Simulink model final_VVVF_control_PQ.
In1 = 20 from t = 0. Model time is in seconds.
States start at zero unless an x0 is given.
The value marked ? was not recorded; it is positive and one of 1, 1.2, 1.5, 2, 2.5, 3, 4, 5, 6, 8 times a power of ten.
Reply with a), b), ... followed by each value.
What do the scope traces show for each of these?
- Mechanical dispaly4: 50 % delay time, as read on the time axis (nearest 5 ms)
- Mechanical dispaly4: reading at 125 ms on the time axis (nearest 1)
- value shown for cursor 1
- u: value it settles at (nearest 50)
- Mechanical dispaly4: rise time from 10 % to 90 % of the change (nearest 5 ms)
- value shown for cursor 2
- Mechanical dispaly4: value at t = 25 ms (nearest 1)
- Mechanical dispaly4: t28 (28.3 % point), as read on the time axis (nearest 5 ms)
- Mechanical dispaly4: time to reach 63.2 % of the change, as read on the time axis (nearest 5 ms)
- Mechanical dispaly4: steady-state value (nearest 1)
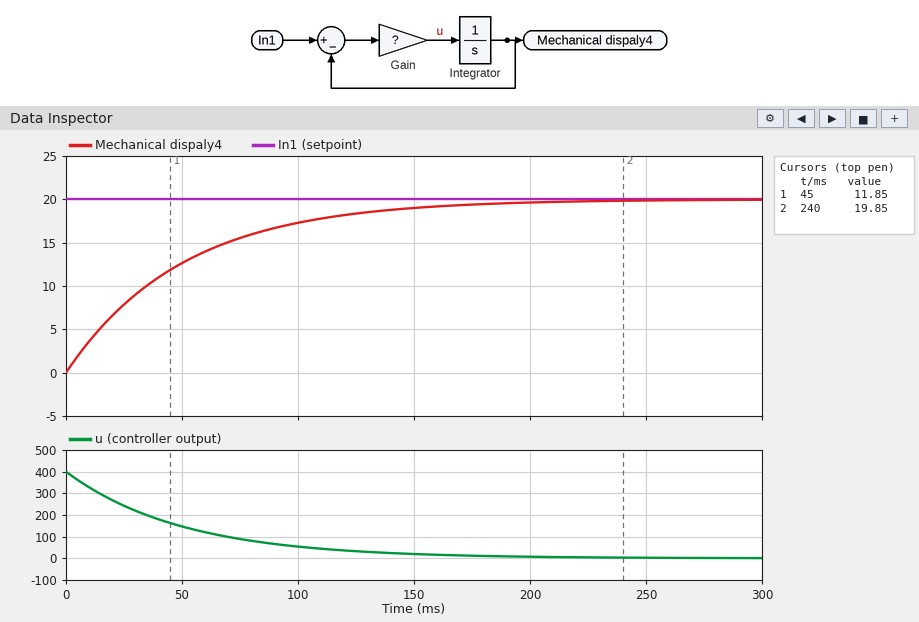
a) 35 ms
b) 18
c) 11.85
d) 0
e) 110 ms
f) 19.85
g) 8
h) 15 ms
i) 50 ms
j) 20
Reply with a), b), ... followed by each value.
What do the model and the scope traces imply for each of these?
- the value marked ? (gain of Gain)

a) 20
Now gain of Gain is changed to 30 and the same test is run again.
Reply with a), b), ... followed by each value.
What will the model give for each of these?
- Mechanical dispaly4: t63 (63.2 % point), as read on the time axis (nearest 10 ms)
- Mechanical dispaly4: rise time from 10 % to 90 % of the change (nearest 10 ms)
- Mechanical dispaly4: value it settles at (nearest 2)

a) 30 ms
b) 70 ms
c) 20
